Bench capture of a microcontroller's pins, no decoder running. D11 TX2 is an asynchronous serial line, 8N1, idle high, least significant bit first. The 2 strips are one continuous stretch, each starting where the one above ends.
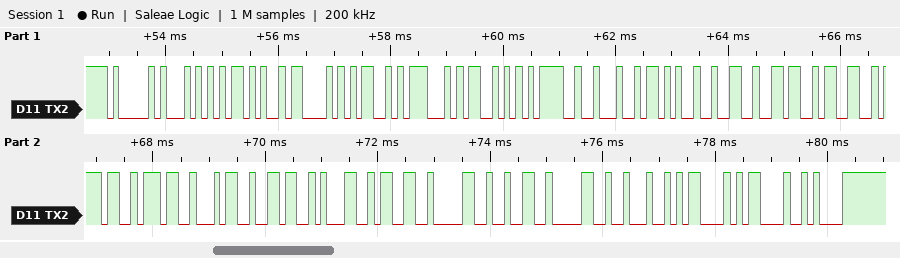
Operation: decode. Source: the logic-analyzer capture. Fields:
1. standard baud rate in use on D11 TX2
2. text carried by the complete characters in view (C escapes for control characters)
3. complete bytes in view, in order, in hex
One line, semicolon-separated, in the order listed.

9600 baud; "AT+CMGS=\"+263774613020\"\r\r\n"; 41 54 2B 43 4D 47 53 3D 22 2B 32 36 33 37 37 34 36 31 33 30 32 30 22 0D 0D 0A
